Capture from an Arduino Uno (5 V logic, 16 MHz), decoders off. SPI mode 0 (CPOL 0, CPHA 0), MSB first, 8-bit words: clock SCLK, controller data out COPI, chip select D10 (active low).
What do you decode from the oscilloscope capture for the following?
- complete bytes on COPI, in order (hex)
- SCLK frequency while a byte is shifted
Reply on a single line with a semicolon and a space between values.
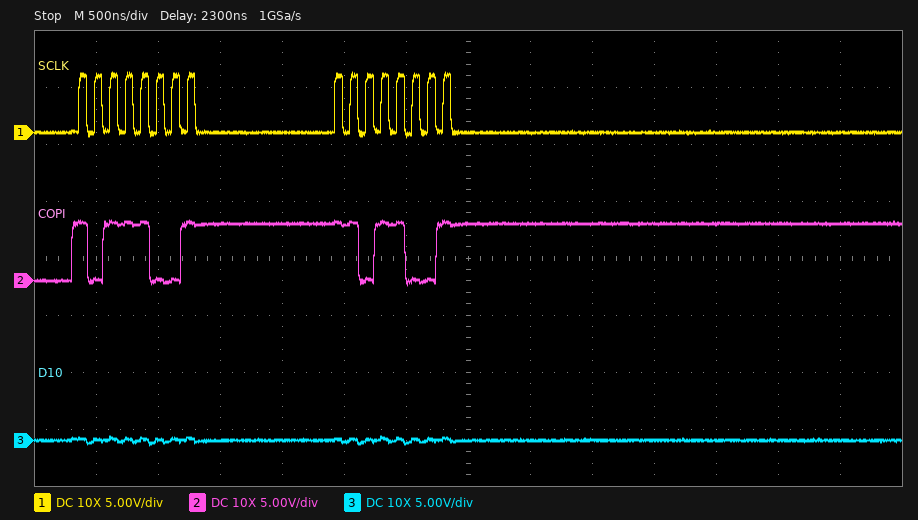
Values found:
B9 D9; 8 MHz
